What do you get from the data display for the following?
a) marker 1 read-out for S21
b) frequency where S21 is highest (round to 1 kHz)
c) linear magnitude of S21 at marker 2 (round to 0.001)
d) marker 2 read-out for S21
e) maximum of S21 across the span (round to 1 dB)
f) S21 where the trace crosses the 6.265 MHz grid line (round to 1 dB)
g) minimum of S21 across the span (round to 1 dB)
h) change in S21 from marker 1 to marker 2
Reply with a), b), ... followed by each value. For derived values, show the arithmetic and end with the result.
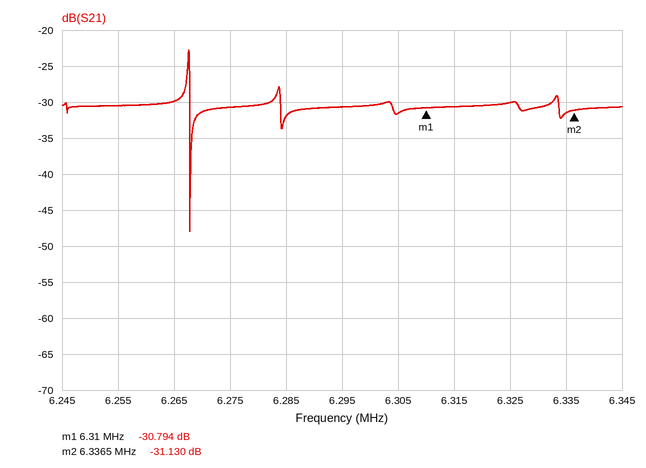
a) -30.794 dB
b) 6.268 MHz
c) 10^(-31.13/20) ≈ 0.028
d) -31.130 dB
e) -23 dB
f) -30 dB
g) -48 dB
h) -31.13 − (-30.794) = -0.336 dB
